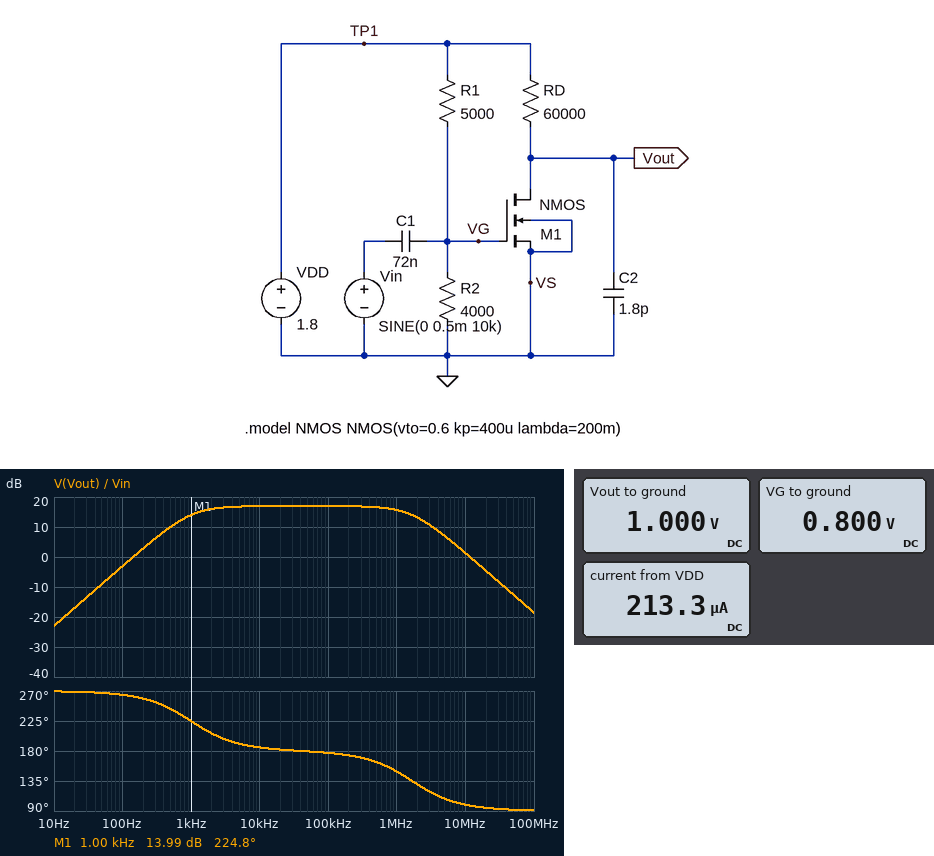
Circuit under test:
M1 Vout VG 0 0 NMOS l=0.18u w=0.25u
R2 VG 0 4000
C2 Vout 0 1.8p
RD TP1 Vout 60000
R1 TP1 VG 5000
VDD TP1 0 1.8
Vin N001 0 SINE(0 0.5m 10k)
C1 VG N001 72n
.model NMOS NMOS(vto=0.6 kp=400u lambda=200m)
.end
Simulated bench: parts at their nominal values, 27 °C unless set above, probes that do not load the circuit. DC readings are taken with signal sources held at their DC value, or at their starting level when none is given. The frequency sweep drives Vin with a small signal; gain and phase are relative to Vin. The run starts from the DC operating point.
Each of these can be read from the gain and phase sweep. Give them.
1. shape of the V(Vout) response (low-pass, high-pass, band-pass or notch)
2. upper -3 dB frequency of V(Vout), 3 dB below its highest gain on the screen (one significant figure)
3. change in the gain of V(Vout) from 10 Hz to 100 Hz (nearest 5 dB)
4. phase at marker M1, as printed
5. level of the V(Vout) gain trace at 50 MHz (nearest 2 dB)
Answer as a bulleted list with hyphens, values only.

- band-pass
- 2 MHz
- 20 dB
- 224.8 deg
- -12 dB
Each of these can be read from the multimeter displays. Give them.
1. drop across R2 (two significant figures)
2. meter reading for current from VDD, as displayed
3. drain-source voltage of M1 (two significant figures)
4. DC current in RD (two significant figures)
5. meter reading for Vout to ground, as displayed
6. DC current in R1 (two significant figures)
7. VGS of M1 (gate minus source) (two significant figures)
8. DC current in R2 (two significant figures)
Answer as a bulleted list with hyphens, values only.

- 800 mV
- 213.3 µA
- 1.0 V
- 13 µA
- 1.000 V
- 200 µA
- 800 mV
- 200 µA
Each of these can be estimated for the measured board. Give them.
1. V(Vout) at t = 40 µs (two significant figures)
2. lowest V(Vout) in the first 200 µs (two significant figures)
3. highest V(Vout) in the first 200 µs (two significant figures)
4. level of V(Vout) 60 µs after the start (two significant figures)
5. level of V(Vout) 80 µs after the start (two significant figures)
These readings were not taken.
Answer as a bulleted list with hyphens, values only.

- 1.0 V
- 1.0 V
- 1.0 V
- 1.0 V
- 1.0 V
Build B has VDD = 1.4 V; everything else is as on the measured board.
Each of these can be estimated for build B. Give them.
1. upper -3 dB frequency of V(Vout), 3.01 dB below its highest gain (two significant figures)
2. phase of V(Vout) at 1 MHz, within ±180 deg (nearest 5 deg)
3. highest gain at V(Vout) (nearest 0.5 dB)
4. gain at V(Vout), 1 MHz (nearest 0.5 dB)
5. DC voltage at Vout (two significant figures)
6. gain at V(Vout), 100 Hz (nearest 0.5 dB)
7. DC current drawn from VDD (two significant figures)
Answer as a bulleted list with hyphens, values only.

- 1.5 MHz
- 145 deg
- -0.5 dB
- -2.0 dB
- 1.4 V
- -20.5 dB
- 160 µA
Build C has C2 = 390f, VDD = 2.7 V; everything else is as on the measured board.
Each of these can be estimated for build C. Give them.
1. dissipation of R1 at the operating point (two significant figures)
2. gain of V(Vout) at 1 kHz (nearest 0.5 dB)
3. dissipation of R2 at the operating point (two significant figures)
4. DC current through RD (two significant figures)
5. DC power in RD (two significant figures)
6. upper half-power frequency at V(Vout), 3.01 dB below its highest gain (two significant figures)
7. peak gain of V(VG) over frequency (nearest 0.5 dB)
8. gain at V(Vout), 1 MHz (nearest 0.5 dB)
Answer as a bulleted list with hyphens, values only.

- 450 µW
- -14.0 dB
- 360 µW
- 43 µA
- 110 µW
- 120 MHz
- 0 dB
- -11.0 dB
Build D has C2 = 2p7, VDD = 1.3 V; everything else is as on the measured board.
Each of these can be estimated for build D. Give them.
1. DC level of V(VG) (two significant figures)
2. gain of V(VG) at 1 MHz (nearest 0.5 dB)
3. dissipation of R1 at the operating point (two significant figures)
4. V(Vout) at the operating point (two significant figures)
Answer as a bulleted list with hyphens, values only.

- 580 mV
- 0 dB
- 100 µW
- 1.3 V
